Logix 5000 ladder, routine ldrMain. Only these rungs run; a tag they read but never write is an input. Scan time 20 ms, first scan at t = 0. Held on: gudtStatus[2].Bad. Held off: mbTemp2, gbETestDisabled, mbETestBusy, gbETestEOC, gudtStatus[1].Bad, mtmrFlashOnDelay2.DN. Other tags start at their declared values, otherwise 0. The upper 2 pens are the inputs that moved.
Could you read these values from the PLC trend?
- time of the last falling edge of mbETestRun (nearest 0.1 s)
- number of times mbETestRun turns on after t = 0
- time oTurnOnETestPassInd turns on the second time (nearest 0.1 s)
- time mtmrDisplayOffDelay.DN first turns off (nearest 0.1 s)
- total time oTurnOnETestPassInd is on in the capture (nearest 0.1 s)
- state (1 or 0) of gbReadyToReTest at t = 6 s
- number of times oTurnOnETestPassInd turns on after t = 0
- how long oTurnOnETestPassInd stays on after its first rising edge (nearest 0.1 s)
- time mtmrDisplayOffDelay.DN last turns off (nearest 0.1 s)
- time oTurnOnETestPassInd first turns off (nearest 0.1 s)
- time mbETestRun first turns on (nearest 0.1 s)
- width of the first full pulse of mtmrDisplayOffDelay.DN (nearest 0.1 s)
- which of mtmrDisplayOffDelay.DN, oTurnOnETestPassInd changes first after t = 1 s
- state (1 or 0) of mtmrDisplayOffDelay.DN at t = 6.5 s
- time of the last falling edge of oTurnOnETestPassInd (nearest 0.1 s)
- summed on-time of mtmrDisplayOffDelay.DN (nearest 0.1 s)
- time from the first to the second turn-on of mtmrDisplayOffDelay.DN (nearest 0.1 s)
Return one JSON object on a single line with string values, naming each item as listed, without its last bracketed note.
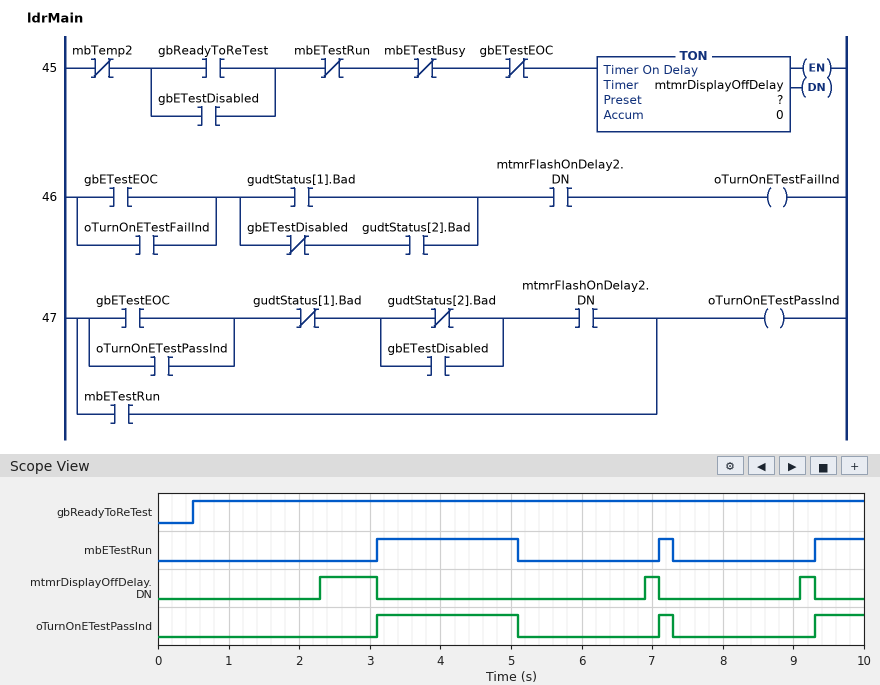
{"time of the last falling edge of mbETestRun": "7.3 s", "number of times mbETestRun turns on after t = 0": "3", "time oTurnOnETestPassInd turns on the second time": "7.1 s", "time mtmrDisplayOffDelay.DN first turns off": "3.1 s", "total time oTurnOnETestPassInd is on in the capture": "2.9 s", "state (1 or 0) of gbReadyToReTest at t = 6 s": "1", "number of times oTurnOnETestPassInd turns on after t = 0": "3", "how long oTurnOnETestPassInd stays on after its first rising edge": "2.0 s", "time mtmrDisplayOffDelay.DN last turns off": "9.3 s", "time oTurnOnETestPassInd first turns off": "5.1 s", "time mbETestRun first turns on": "3.1 s", "width of the first full pulse of mtmrDisplayOffDelay.DN": "0.8 s", "which of mtmrDisplayOffDelay.DN, oTurnOnETestPassInd changes first after t = 1 s": "mtmrDisplayOffDelay.DN", "state (1 or 0) of mtmrDisplayOffDelay.DN at t = 6.5 s": "0", "time of the last falling edge of oTurnOnETestPassInd": "7.3 s", "summed on-time of mtmrDisplayOffDelay.DN": "1.2 s", "time from the first to the second turn-on of mtmrDisplayOffDelay.DN": "4.6 s"}
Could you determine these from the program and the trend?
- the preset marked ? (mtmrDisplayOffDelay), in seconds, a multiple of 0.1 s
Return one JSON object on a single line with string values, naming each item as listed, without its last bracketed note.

{"the preset marked ? (mtmrDisplayOffDelay), in seconds, a multiple of 0.1 s": "1.8 s"}
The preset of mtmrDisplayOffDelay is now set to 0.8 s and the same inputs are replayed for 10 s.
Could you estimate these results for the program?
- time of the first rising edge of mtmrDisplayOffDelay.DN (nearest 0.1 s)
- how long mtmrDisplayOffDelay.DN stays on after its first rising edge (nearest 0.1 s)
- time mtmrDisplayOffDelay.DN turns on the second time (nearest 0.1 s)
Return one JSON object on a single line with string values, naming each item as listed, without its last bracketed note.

{"time of the first rising edge of mtmrDisplayOffDelay.DN": "1.3 s", "how long mtmrDisplayOffDelay.DN stays on after its first rising edge": "1.8 s", "time mtmrDisplayOffDelay.DN turns on the second time": "5.9 s"}
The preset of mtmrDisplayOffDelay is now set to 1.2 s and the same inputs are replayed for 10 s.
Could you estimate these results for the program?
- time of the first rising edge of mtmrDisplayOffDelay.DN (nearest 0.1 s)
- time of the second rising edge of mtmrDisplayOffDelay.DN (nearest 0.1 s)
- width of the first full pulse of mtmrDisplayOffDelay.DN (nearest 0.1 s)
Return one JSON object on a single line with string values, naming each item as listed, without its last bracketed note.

{"time of the first rising edge of mtmrDisplayOffDelay.DN": "1.7 s", "time of the second rising edge of mtmrDisplayOffDelay.DN": "6.3 s", "width of the first full pulse of mtmrDisplayOffDelay.DN": "1.4 s"}
